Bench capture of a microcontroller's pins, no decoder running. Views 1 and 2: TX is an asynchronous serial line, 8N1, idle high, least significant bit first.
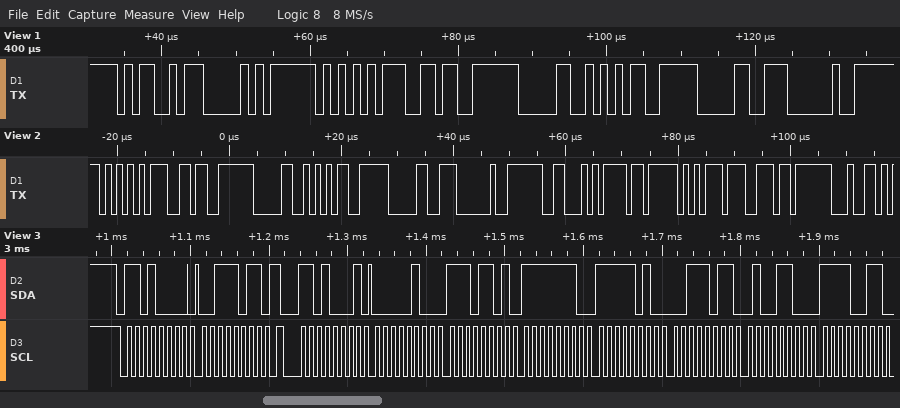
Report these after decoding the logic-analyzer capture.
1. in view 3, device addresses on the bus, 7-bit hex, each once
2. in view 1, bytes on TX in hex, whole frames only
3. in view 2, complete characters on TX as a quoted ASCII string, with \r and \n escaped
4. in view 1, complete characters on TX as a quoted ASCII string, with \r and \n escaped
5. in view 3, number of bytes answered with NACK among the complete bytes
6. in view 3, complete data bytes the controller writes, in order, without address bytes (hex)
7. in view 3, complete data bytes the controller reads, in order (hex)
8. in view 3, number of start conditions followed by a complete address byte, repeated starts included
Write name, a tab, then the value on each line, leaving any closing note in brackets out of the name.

in view 3, device addresses on the bus, 7-bit hex, each once	0x68
in view 1, bytes on TX in hex, whole frames only	0x4D 0x50 0x55 0x36 0x30 0x35 0x30 0x20
in view 2, complete characters on TX as a quoted ASCII string, with \r and \n escaped	"U6050 Found"
in view 1, complete characters on TX as a quoted ASCII string, with \r and \n escaped	"MPU6050 "
in view 3, number of bytes answered with NACK among the complete bytes	0
in view 3, complete data bytes the controller writes, in order, without address bytes	3B
in view 3, complete data bytes the controller reads, in order	04 ED FE FA 3B 4C F3
in view 3, number of start conditions followed by a complete address byte, repeated starts included	2
